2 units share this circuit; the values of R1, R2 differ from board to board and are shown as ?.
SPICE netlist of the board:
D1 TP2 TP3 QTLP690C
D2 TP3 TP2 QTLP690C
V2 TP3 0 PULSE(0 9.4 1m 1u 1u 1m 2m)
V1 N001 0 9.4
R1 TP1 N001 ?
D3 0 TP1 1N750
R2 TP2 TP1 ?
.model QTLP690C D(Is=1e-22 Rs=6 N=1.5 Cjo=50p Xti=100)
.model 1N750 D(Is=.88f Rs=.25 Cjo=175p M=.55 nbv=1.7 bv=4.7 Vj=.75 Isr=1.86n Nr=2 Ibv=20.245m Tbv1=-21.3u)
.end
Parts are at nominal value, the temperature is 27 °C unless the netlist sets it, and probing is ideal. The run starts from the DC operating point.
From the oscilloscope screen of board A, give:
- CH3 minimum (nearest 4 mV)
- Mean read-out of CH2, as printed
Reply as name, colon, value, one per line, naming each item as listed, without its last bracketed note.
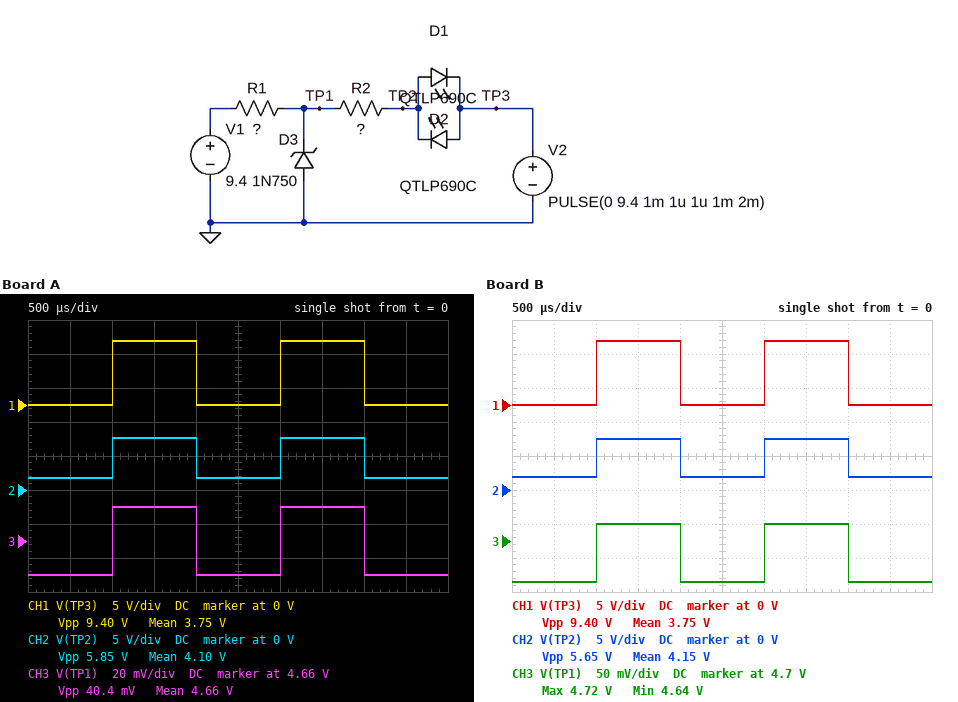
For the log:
CH3 minimum: 4.640 V
Mean read-out of CH2, as printed: 4.10 V
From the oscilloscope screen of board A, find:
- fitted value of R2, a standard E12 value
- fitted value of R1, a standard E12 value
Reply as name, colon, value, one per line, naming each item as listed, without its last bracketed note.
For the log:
fitted value of R2, a standard E12 value: 820 Ω
fitted value of R1, a standard E12 value: 560 Ω
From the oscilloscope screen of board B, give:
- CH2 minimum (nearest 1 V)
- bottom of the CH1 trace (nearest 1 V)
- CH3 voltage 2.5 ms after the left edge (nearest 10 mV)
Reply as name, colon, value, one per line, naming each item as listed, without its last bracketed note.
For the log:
CH2 minimum: 2 V
bottom of the CH1 trace: 0 V
CH3 voltage 2.5 ms after the left edge: 4.64 V
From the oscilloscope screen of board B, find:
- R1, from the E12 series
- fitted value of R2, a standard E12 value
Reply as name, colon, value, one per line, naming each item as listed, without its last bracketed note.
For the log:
R1, from the E12 series: 270 Ω
fitted value of R2, a standard E12 value: 220 Ω
